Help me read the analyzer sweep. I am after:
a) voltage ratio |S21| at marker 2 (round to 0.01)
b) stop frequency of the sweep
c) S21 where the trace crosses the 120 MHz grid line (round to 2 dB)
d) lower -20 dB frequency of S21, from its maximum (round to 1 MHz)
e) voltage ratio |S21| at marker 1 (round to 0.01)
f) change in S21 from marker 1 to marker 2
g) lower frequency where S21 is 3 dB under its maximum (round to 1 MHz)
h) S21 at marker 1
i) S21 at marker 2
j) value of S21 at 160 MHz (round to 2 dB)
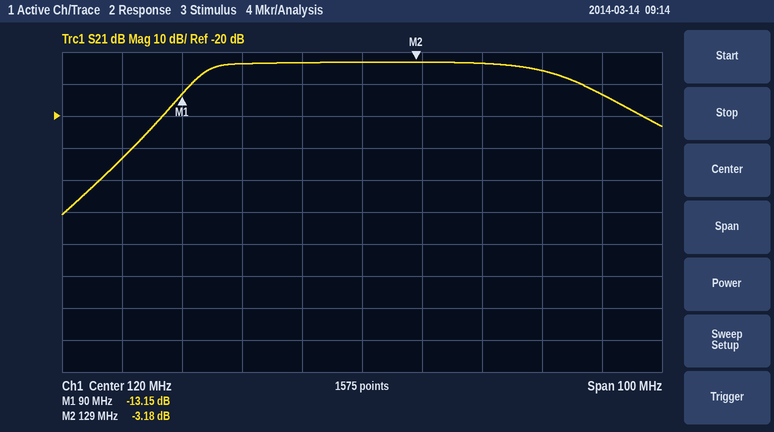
0.69
170 MHz
-4 dB
85 MHz
0.22
9.97 dB
94 MHz
-13.15 dB
-3.18 dB
-14 dB
